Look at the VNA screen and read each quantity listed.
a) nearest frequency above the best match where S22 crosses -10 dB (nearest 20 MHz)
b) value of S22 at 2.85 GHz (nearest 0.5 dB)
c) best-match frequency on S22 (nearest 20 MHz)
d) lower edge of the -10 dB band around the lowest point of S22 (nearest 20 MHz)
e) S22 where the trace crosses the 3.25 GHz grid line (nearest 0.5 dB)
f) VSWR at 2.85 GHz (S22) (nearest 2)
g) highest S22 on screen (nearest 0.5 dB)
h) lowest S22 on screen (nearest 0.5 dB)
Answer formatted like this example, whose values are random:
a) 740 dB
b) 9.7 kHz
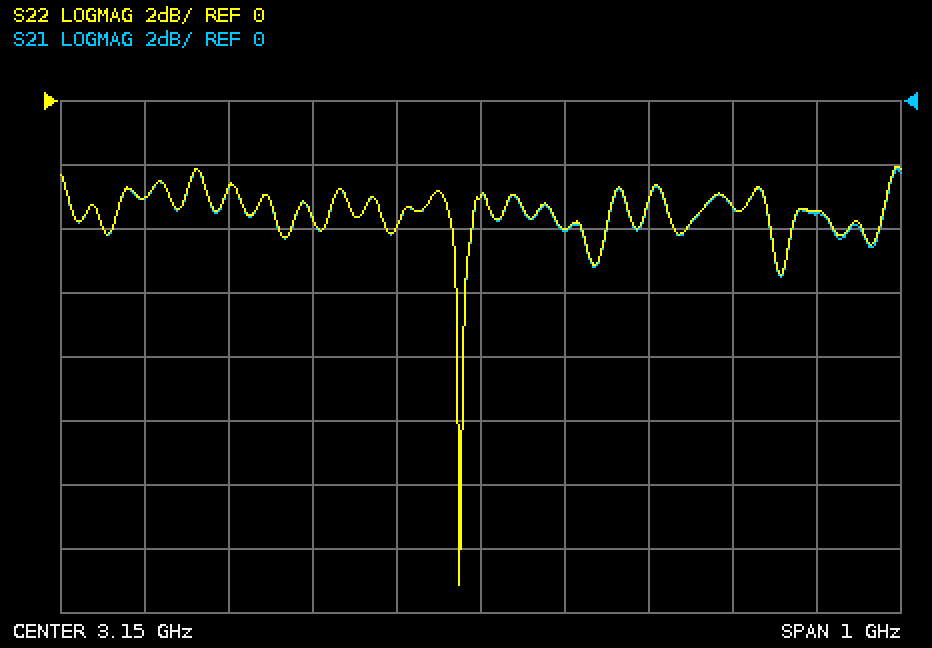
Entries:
a) 3.12 GHz
b) -2.5 dB
c) 3.12 GHz
d) 3.12 GHz
e) -4.0 dB
f) 6
g) -2.0 dB
h) -15.0 dB
